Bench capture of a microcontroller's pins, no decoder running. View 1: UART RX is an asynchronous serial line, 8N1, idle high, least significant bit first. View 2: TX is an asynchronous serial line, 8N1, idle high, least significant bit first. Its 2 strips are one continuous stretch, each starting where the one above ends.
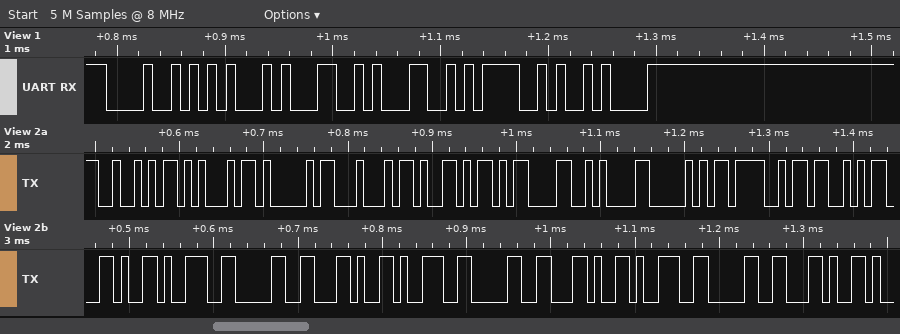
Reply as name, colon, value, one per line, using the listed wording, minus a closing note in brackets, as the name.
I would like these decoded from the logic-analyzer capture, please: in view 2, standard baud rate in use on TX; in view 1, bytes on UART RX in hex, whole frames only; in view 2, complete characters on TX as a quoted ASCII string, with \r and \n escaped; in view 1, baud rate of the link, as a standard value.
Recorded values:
in view 2, standard baud rate in use on TX: 115200 baud
in view 1, bytes on UART RX in hex, whole frames only: 0x48 0x45 0x4C 0x4C 0x4F 0x0A
in view 2, complete characters on TX as a quoted ASCII string, with \r and \n escaped: "READY\r\nPOS,90,90,90,"
in view 1, baud rate of the link, as a standard value: 115200 baud
